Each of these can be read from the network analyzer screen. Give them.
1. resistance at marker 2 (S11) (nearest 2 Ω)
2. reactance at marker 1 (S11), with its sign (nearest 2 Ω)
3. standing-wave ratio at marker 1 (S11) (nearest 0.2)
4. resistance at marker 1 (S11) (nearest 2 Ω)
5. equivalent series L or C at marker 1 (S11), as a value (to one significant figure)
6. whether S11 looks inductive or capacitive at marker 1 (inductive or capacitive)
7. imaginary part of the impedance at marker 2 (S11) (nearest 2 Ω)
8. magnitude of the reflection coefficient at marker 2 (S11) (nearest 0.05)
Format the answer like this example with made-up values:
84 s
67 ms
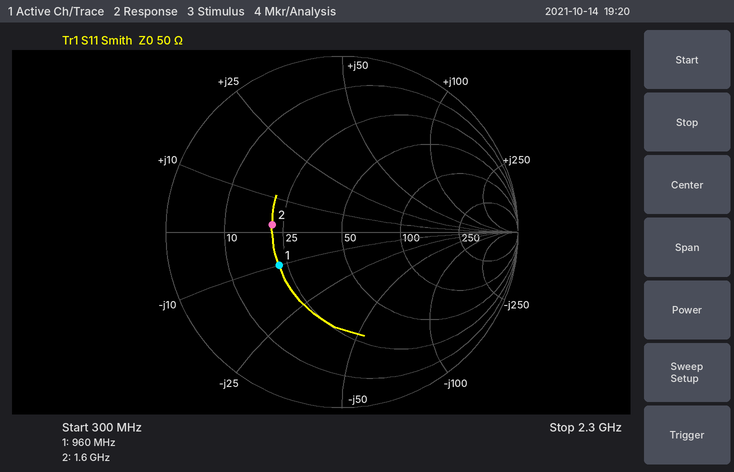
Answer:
22 Ω
-10 Ω
2.4
22 Ω
20 pF
capacitive
+2 Ω
0.40
